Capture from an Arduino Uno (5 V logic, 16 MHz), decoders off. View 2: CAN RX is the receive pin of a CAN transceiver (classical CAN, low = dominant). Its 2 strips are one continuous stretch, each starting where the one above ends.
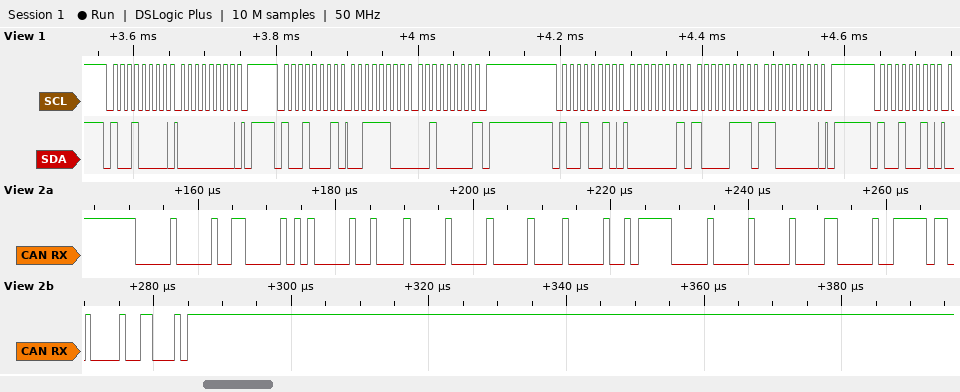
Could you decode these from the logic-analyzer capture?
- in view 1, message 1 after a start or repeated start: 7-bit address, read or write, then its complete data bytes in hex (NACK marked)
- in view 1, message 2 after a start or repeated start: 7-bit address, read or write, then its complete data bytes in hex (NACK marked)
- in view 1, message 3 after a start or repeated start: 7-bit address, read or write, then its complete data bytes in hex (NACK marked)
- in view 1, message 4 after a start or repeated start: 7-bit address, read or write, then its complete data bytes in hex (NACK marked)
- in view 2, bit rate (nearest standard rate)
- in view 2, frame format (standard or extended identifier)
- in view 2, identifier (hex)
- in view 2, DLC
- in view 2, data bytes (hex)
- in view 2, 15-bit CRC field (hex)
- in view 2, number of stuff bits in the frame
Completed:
0x48 write: 00
0x48 read: 3C 20 NACK
0x49 write: 01 87 C0
0x49 write
1000 kbit/s
extended
0x00000A02
8
00 00 80 BE 00 00 60 3F
0x5098
14
